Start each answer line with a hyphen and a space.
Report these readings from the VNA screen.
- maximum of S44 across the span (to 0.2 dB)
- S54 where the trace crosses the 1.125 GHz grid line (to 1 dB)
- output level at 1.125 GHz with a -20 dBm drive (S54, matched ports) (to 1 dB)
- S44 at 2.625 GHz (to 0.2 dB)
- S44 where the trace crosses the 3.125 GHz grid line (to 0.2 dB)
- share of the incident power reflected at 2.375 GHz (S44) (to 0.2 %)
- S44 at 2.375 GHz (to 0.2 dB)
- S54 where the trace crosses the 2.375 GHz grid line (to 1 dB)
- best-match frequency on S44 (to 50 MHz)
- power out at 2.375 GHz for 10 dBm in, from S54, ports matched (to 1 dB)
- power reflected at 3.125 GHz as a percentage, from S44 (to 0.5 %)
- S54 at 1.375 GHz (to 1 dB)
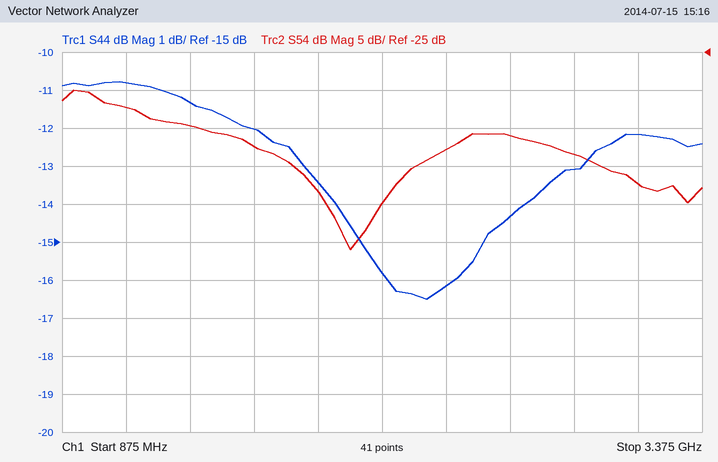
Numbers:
- -10.8 dB
- -32 dB
- -52 dBm
- -14.4 dB
- -12.2 dB
- 2.4 %
- -16.2 dB
- -38 dB
- 2.30 GHz
- -28 dBm
- 6.0 %
- -35 dB
